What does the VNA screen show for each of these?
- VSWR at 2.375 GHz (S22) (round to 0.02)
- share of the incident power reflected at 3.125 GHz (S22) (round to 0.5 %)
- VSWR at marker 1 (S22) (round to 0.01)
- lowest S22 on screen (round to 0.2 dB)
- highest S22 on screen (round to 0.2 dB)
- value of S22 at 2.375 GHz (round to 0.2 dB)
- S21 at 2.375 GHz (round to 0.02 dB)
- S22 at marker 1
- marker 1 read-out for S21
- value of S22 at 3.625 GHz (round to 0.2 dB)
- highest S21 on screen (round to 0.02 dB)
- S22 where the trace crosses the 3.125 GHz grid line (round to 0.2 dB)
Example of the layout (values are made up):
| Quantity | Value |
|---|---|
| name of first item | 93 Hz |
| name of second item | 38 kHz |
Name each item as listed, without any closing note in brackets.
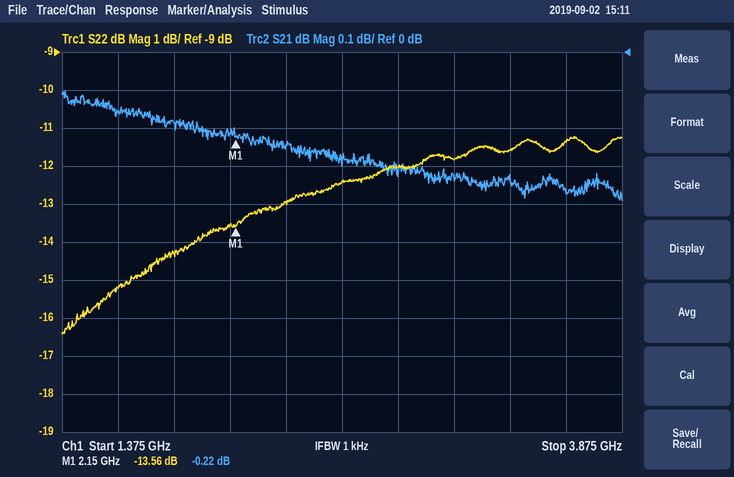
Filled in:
| Quantity | Value |
|---|---|
| VSWR at 2.375 GHz (S22) | 1.58 |
| share of the incident power reflected at 3.125 GHz (S22) | 6.5 % |
| VSWR at marker 1 (S22) | 1.53 |
| lowest S22 on screen | -16.4 dB |
| highest S22 on screen | -11.2 dB |
| value of S22 at 2.375 GHz | -13.0 dB |
| S21 at 2.375 GHz | -0.24 dB |
| S22 at marker 1 | -13.56 dB |
| marker 1 read-out for S21 | -0.22 dB |
| value of S22 at 3.625 GHz | -11.4 dB |
| highest S21 on screen | -0.10 dB |
| S22 where the trace crosses the 3.125 GHz grid line | -11.8 dB |
